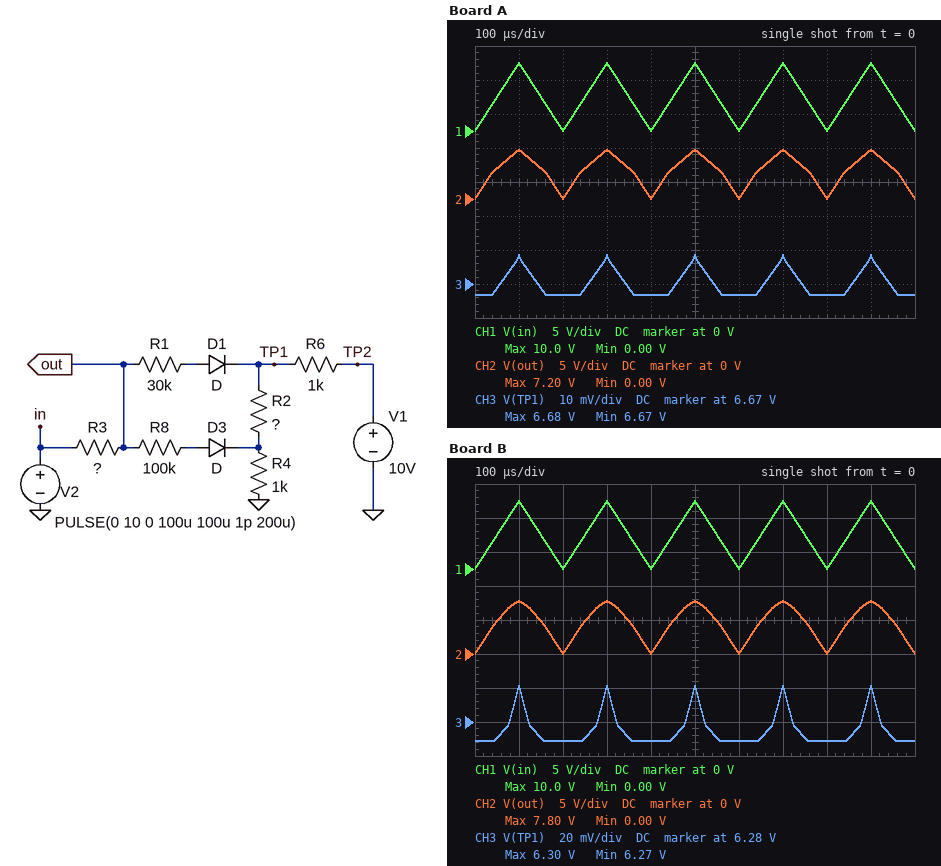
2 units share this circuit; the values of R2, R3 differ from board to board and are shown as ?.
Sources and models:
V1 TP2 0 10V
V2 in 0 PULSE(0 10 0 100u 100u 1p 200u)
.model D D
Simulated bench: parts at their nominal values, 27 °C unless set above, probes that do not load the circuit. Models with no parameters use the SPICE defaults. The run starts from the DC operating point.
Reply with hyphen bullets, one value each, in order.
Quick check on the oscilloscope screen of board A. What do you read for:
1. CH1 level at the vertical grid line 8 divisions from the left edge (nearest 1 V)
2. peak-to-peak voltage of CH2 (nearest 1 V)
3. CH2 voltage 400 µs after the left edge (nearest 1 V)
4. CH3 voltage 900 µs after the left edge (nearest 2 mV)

- 0 V
- 7 V
- 0 V
- 6.678 V
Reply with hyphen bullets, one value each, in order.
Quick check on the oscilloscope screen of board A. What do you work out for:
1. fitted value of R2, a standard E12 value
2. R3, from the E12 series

- 1 kΩ
- 82 kΩ
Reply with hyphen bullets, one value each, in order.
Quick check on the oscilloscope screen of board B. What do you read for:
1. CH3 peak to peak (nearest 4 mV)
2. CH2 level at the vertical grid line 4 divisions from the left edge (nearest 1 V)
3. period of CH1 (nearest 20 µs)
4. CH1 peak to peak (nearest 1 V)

- 32 mV
- 0 V
- 200 µs
- 10 V
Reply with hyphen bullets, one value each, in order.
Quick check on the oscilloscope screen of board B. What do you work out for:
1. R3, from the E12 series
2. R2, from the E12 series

- 33 kΩ
- 680 Ω
